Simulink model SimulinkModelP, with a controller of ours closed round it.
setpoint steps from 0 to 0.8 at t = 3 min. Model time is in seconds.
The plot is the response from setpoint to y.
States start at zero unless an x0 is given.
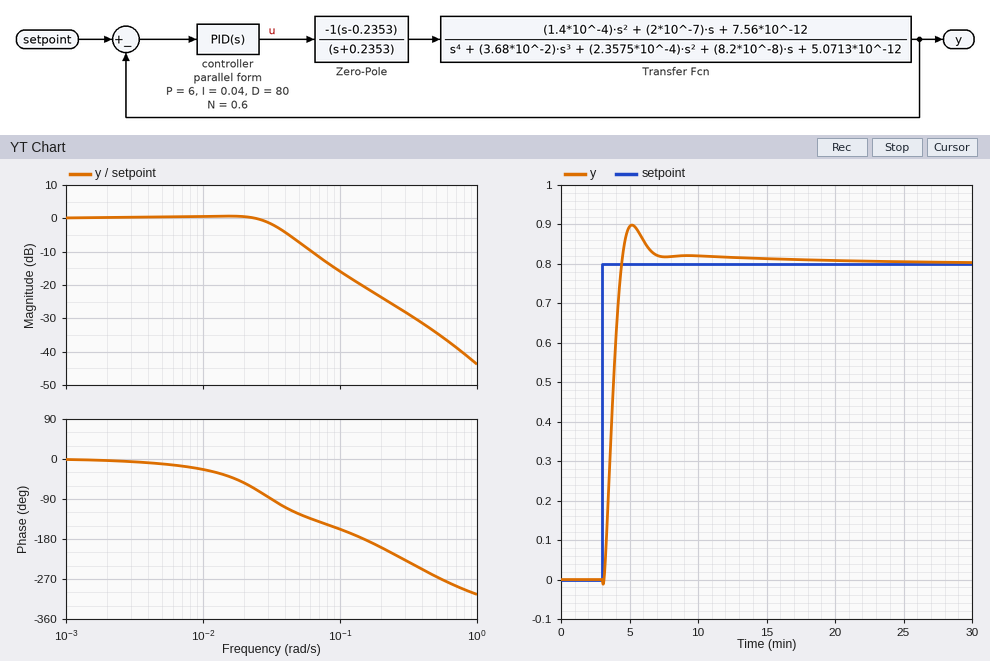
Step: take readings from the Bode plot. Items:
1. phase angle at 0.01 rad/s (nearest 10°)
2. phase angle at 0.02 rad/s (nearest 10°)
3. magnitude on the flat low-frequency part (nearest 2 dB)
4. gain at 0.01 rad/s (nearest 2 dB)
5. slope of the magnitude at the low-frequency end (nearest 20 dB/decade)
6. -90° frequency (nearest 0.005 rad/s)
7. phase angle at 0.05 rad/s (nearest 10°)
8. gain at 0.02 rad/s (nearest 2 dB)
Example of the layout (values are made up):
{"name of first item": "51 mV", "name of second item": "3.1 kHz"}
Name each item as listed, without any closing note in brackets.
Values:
{"phase angle at 0.01 rad/s": "-20°", "phase angle at 0.02 rad/s": "-50°", "magnitude on the flat low-frequency part": "0 dB", "gain at 0.01 rad/s": "0 dB", "slope of the magnitude at the low-frequency end": "0 dB/decade", "-90° frequency": "0.030 rad/s", "phase angle at 0.05 rad/s": "-120°", "gain at 0.02 rad/s": "0 dB"}
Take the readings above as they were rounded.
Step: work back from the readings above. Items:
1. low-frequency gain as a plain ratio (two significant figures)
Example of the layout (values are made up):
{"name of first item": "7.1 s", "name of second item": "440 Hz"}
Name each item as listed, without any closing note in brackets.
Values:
{"low-frequency gain as a plain ratio": "1.0"}
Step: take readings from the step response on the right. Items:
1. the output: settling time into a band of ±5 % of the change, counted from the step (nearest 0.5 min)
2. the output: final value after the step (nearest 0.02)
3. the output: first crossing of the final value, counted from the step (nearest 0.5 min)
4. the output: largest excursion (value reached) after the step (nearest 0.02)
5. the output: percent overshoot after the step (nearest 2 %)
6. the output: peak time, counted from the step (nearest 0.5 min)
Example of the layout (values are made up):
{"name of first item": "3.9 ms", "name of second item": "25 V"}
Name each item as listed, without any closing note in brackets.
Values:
{"the output: settling time into a band of ±5 % of the change, counted from the step": "3.5 min", "the output: final value after the step": "0.80", "the output: first crossing of the final value, counted from the step": "1.5 min", "the output: largest excursion (value reached) after the step": "0.90", "the output: percent overshoot after the step": "12 %", "the output: peak time, counted from the step": "2.0 min"}
